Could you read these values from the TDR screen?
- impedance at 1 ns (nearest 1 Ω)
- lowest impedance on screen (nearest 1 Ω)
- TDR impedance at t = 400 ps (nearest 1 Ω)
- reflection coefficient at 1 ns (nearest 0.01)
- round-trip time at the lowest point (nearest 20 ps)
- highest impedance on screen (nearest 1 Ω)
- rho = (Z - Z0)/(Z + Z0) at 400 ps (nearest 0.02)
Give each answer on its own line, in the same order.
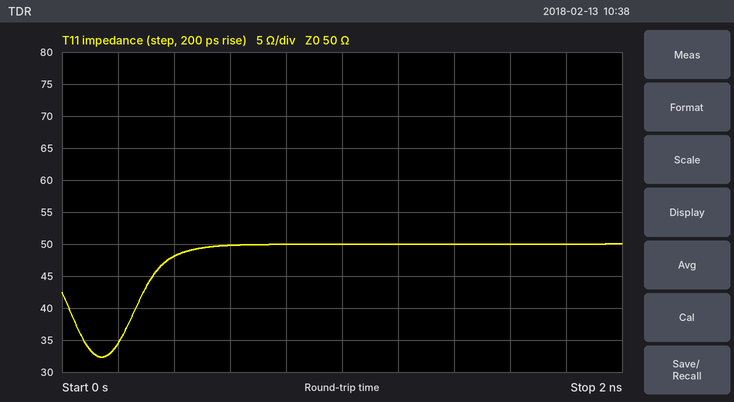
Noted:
50 Ω
32 Ω
48 Ω
0.00
140 ps
50 Ω
-0.02
